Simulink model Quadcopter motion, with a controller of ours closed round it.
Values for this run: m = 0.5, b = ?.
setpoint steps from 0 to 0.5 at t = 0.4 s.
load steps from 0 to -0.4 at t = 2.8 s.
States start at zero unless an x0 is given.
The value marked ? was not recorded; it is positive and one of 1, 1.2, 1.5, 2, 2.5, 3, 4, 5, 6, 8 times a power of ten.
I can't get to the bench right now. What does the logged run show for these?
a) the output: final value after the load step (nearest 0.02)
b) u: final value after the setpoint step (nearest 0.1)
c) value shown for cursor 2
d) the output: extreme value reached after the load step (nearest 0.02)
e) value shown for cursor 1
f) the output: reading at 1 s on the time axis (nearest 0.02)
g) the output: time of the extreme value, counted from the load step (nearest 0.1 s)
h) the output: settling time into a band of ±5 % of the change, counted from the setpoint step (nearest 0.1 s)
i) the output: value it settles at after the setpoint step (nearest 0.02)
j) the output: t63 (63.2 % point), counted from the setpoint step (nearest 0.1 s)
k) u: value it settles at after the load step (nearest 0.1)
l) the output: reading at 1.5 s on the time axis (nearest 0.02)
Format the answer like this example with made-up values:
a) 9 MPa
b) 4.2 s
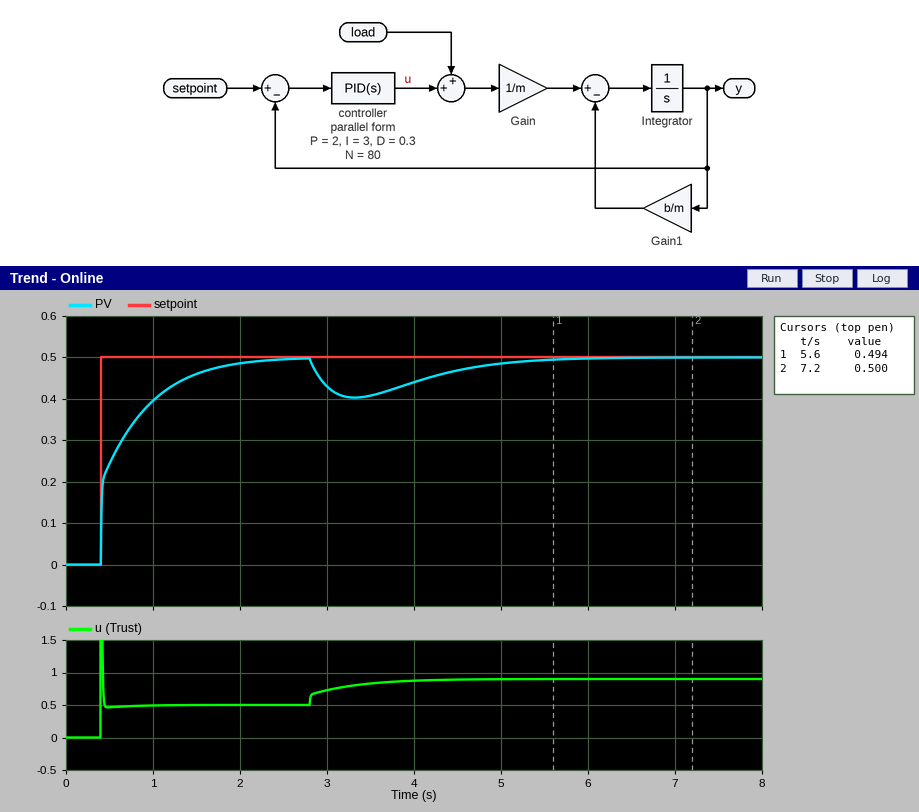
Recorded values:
a) 0.50
b) 0.5
c) 0.500
d) 0.40
e) 0.494
f) 0.40
g) 0.5 s
h) 1.3 s
i) 0.50
j) 0.3 s
k) 0.9
l) 0.46
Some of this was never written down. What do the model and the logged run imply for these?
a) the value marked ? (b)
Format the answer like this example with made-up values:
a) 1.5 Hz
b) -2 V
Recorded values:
a) 1
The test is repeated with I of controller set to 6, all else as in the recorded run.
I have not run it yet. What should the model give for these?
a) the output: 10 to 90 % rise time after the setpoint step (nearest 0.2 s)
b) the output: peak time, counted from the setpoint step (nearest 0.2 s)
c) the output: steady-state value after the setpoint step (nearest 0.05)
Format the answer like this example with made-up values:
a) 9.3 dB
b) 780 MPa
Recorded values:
a) 0.6 s
b) 1.2 s
c) 0.50
